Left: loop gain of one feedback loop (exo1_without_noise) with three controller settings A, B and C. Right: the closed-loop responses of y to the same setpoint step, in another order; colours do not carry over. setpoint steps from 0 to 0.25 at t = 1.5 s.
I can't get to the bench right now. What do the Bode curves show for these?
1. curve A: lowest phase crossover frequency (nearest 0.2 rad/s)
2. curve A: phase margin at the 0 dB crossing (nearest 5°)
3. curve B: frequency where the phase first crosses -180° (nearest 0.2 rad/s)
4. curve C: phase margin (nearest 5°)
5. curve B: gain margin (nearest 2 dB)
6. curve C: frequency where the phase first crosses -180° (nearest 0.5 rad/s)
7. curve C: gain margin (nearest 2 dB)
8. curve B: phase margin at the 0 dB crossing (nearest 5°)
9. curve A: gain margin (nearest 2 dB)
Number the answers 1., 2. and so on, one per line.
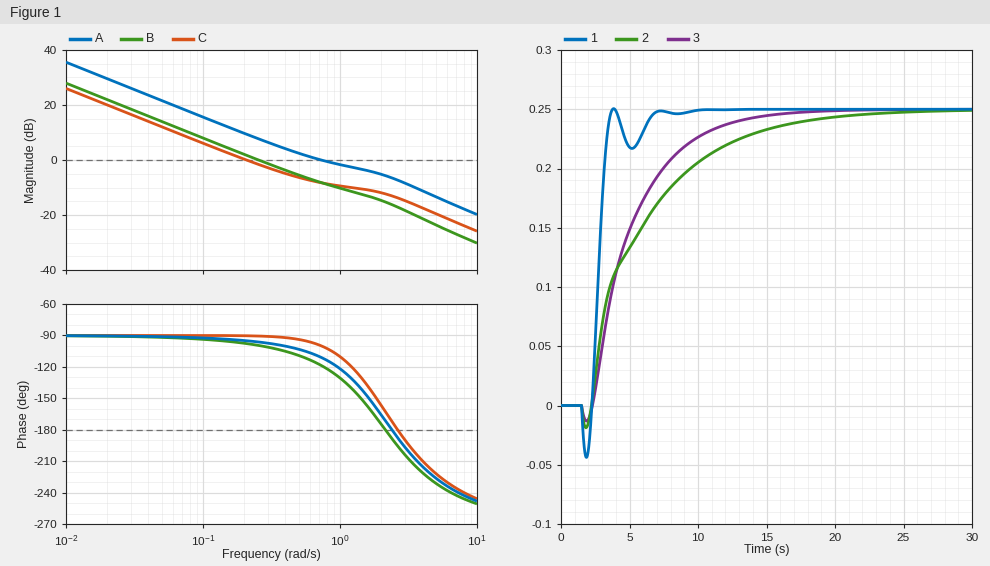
1. 2.4 rad/s
2. 70°
3. 2.2 rad/s
4. 90°
5. 16 dB
6. 2.5 rad/s
7. 14 dB
8. 80°
9. 6 dB
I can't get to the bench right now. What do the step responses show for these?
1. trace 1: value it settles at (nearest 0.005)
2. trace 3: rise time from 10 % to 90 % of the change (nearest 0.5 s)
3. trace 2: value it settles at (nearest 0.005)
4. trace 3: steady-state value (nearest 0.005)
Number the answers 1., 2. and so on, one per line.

1. 0.250
2. 7.0 s
3. 0.250
4. 0.250
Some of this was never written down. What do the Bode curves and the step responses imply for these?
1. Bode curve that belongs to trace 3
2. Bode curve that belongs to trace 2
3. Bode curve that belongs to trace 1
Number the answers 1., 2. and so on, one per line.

1. B
2. C
3. A
